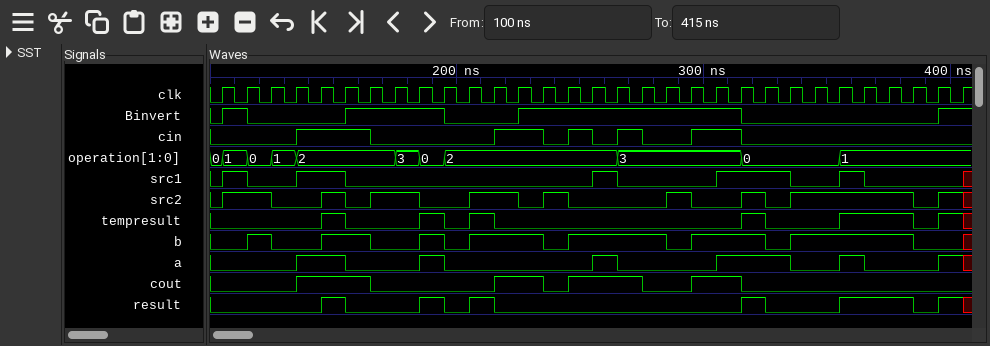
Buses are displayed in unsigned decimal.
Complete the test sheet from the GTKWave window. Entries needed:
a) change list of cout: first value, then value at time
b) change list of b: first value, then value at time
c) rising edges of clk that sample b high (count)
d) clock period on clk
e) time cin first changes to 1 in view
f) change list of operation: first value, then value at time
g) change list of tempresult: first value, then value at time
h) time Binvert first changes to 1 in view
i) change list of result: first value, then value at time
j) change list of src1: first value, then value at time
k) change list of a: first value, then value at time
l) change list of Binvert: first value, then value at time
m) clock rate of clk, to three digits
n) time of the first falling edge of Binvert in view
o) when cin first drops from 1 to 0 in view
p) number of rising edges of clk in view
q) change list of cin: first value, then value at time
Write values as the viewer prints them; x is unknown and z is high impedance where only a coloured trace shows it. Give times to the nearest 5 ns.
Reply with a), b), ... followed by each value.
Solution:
a) 0, 1 at 135 ns, 0 at 165 ns, 1 at 215 ns, 0 at 235 ns, 1 at 245 ns, 0 at 275 ns, 1 at 295 ns, 0 at 315 ns
b) 0, 1 at 115 ns, 0 at 125 ns, 1 at 145 ns, 0 at 165 ns, 1 at 185 ns, 0 at 195 ns, 1 at 205 ns, 0 at 235 ns, 1 at 245 ns, 0 at 285 ns, 1 at 295 ns, 0 at 325 ns, 1 at 335 ns, 0 at 385 ns, x at 405 ns
c) 19
d) 10 ns
e) 135 ns
f) 0, 1 at 105 ns, 0 at 115 ns, 1 at 125 ns, 2 at 135 ns, 3 at 175 ns, 0 at 185 ns, 2 at 195 ns, 3 at 265 ns, 0 at 315 ns, 1 at 355 ns
g) 0, 1 at 145 ns, 0 at 155 ns, 1 at 185 ns, 0 at 195 ns, 1 at 205 ns, 0 at 215 ns, 1 at 315 ns, 0 at 325 ns, 1 at 355 ns, 0 at 385 ns, 1 at 395 ns, x at 405 ns
h) 105 ns
i) 0, 1 at 145 ns, 0 at 155 ns, 1 at 185 ns, 0 at 195 ns, 1 at 205 ns, 0 at 215 ns, 1 at 315 ns, 0 at 325 ns, 1 at 355 ns, 0 at 385 ns, 1 at 395 ns, x at 405 ns
j) 0, 1 at 105 ns, 0 at 115 ns, 1 at 135 ns, 0 at 155 ns, 1 at 255 ns, 0 at 265 ns, 1 at 305 ns, 0 at 335 ns, 1 at 355 ns, 0 at 365 ns, x at 405 ns
k) 0, 1 at 135 ns, 0 at 155 ns, 1 at 185 ns, 0 at 195 ns, 1 at 255 ns, 0 at 265 ns, 1 at 305 ns, 0 at 335 ns, 1 at 355 ns, 0 at 365 ns, 1 at 395 ns, x at 405 ns
l) 0, 1 at 105 ns, 0 at 115 ns, 1 at 155 ns, 0 at 195 ns, 1 at 225 ns, 0 at 315 ns, 1 at 395 ns
m) 100 MHz
n) 115 ns
o) 165 ns
p) 31
q) 0, 1 at 135 ns, 0 at 165 ns, 1 at 215 ns, 0 at 235 ns, 1 at 245 ns, 0 at 255 ns, 1 at 265 ns, 0 at 275 ns, 1 at 295 ns, 0 at 315 ns
